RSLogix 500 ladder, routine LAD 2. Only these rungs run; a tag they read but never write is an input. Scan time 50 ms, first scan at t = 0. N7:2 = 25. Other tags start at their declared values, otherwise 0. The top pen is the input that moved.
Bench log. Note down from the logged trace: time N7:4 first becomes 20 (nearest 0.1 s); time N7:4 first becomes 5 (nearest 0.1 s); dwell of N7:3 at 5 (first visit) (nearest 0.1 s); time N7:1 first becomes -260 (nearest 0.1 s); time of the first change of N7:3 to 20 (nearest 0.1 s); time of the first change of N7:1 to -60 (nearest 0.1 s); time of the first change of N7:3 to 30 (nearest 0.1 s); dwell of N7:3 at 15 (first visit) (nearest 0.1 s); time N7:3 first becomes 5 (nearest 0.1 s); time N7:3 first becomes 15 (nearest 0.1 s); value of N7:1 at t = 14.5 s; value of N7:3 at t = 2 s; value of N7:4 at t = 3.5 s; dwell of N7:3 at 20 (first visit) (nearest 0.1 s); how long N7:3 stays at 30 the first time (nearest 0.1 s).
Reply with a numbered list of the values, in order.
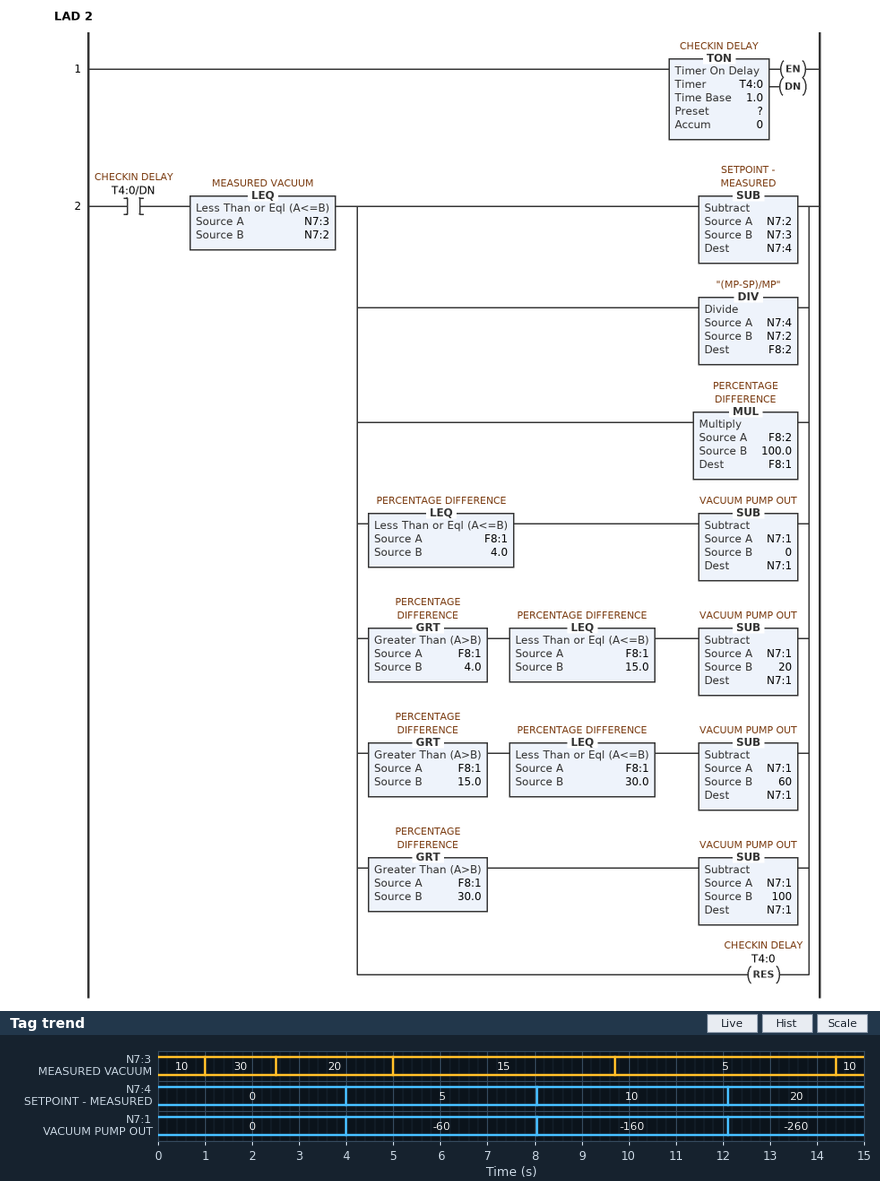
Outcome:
1. 12.1 s
2. 4.0 s
3. 4.7 s
4. 12.1 s
5. 2.5 s
6. 4.0 s
7. 1.0 s
8. 4.7 s
9. 9.7 s
10. 5.0 s
11. -260
12. 30
13. 0
14. 2.5 s
15. 1.5 s
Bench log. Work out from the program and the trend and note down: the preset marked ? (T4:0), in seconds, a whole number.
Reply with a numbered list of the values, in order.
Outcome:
1. 4 s
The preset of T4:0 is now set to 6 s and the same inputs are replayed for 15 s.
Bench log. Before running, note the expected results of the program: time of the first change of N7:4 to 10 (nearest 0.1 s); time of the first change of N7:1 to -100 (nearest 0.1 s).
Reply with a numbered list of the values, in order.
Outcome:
1. 6.0 s
2. 6.0 s
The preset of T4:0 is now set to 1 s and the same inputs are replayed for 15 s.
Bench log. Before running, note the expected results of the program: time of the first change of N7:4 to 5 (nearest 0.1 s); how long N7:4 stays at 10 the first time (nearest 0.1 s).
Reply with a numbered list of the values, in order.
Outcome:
1. 2.5 s
2. 4.2 s
